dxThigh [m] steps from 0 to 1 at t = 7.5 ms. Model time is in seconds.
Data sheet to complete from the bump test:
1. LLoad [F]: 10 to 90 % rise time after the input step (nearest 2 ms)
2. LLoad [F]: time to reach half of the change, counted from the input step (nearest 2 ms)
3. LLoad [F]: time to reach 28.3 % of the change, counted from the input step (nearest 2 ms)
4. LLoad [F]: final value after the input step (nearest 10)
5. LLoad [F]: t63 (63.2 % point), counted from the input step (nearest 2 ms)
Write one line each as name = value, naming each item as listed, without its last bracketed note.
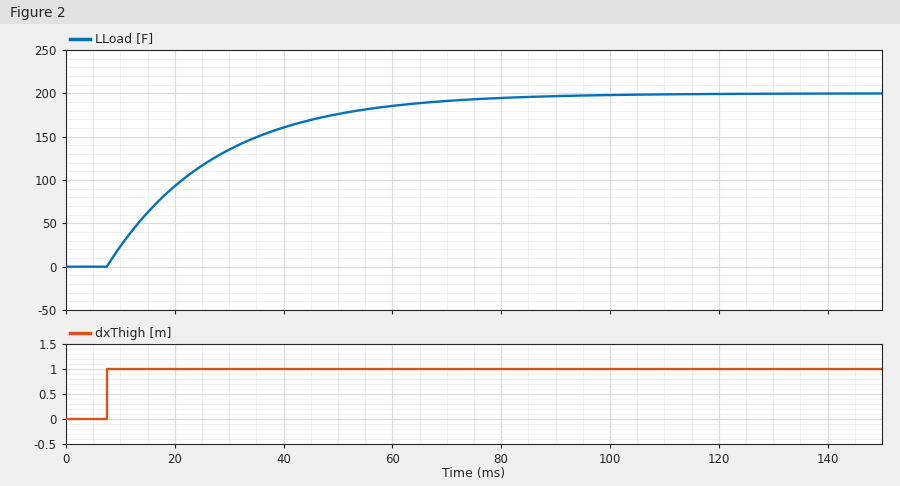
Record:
LLoad [F]: 10 to 90 % rise time after the input step = 44 ms
LLoad [F]: time to reach half of the change, counted from the input step = 14 ms
LLoad [F]: time to reach 28.3 % of the change, counted from the input step = 6 ms
LLoad [F]: final value after the input step = 200
LLoad [F]: t63 (63.2 % point), counted from the input step = 20 ms
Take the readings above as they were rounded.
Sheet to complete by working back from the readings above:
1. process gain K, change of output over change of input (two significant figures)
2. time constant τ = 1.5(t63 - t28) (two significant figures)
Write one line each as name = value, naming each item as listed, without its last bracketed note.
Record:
process gain K, change of output over change of input = 200
time constant τ = 1.5(t63 - t28) = 21 ms
